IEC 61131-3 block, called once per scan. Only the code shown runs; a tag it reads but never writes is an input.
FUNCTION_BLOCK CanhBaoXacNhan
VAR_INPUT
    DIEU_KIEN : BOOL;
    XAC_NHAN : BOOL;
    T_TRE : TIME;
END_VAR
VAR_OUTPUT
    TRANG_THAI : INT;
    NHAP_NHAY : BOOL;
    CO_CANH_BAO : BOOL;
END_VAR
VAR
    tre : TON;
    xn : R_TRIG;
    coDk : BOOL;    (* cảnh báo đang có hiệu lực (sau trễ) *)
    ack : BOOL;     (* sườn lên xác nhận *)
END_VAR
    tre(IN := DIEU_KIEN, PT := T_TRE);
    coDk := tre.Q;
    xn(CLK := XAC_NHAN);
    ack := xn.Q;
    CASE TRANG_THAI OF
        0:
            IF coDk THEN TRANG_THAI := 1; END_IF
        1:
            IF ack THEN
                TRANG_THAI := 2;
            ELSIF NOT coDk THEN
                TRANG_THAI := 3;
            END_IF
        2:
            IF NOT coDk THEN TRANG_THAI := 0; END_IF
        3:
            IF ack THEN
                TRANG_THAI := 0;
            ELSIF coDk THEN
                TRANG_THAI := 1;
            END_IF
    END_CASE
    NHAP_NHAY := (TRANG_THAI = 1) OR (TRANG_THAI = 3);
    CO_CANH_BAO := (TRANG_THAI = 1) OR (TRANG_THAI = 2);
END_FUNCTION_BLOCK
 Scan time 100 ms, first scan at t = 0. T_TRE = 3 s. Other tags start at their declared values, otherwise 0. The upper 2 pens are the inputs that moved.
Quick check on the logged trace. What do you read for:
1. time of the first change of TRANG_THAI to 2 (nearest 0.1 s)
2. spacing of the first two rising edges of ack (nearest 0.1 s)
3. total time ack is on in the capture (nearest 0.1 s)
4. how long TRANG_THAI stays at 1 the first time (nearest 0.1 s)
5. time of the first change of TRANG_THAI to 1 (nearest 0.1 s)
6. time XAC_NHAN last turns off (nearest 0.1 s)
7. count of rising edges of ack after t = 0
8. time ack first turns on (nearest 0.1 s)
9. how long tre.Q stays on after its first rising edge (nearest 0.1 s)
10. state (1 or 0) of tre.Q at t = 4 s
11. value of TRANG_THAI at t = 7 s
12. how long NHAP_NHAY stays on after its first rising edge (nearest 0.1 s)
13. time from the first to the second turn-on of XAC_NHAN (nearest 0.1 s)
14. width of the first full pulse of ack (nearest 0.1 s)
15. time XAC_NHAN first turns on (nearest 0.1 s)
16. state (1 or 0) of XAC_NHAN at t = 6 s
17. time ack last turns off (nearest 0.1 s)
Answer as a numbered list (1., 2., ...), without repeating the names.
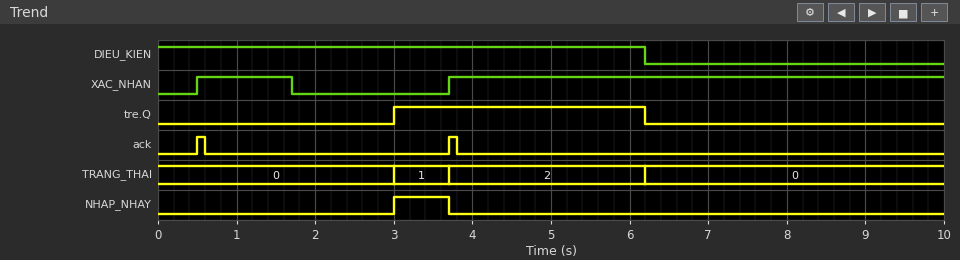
1. 3.7 s
2. 3.2 s
3. 0.2 s
4. 0.7 s
5. 3.0 s
6. 1.7 s
7. 2
8. 0.5 s
9. 3.2 s
10. 1
11. 0
12. 0.7 s
13. 3.2 s
14. 0.1 s
15. 0.5 s
16. 1
17. 3.8 s
